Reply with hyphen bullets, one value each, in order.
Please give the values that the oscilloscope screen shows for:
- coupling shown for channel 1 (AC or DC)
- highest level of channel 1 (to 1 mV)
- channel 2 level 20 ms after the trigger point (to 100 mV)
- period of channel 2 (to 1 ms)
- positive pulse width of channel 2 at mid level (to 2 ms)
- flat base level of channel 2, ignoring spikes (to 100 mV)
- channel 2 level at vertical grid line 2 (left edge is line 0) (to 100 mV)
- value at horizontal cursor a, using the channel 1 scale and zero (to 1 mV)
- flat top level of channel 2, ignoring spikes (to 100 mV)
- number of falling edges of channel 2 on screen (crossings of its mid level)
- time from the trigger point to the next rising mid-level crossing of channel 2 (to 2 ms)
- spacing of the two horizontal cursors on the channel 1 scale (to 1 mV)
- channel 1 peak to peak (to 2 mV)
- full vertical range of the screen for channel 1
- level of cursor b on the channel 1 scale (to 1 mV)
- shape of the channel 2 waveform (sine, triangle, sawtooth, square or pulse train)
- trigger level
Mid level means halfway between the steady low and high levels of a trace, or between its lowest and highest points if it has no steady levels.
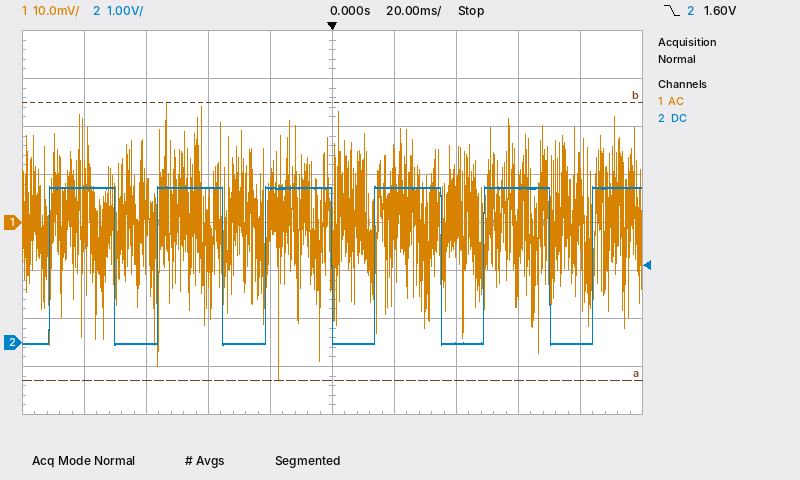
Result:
- AC
- 25 mV
- 3.2 V
- 35 ms
- 22 ms
- 0.0 V
- 0.0 V
- -33 mV
- 3.2 V
- 5
- 14 ms
- 58 mV
- 58 mV
- 80 mV
- 25 mV
- pulse train
- 1.60 V
